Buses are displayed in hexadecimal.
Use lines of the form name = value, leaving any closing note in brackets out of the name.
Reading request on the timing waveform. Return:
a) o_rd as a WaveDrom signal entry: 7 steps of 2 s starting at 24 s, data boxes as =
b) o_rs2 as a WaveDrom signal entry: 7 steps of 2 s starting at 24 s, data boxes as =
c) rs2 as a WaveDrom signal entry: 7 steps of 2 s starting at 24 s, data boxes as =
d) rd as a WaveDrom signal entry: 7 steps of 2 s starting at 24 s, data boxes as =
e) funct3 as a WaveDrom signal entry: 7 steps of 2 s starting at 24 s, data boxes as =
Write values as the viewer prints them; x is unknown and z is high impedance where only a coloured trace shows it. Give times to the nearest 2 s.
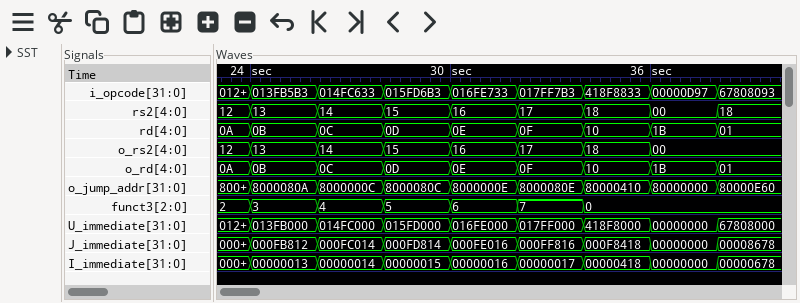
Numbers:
o_rd as a WaveDrom signal entry: 7 steps of 2 s starting at 24 s, data boxes as = = {name: 'o_rd', wave: '=======', data: '0B 0C 0D 0E 0F 10 1B'}
o_rs2 as a WaveDrom signal entry: 7 steps of 2 s starting at 24 s, data boxes as = = {name: 'o_rs2', wave: '=======', data: '13 14 15 16 17 18 00'}
rs2 as a WaveDrom signal entry: 7 steps of 2 s starting at 24 s, data boxes as = = {name: 'rs2', wave: '=======', data: '13 14 15 16 17 18 00'}
rd as a WaveDrom signal entry: 7 steps of 2 s starting at 24 s, data boxes as = = {name: 'rd', wave: '=======', data: '0B 0C 0D 0E 0F 10 1B'}
funct3 as a WaveDrom signal entry: 7 steps of 2 s starting at 24 s, data boxes as = = {name: 'funct3', wave: '======.', data: '3 4 5 6 7 0'}
